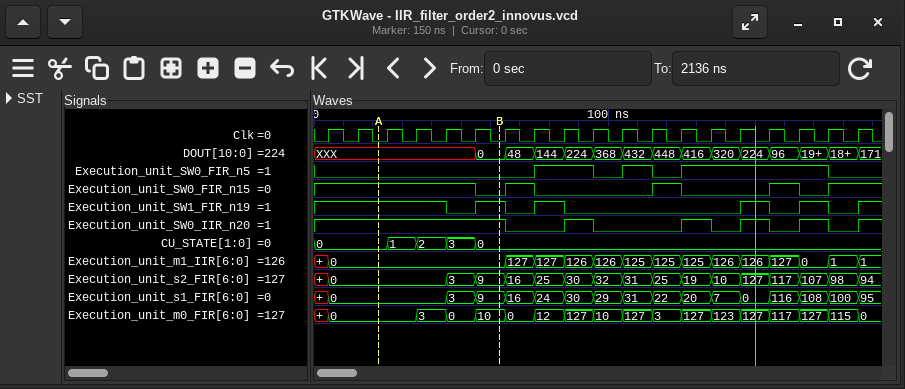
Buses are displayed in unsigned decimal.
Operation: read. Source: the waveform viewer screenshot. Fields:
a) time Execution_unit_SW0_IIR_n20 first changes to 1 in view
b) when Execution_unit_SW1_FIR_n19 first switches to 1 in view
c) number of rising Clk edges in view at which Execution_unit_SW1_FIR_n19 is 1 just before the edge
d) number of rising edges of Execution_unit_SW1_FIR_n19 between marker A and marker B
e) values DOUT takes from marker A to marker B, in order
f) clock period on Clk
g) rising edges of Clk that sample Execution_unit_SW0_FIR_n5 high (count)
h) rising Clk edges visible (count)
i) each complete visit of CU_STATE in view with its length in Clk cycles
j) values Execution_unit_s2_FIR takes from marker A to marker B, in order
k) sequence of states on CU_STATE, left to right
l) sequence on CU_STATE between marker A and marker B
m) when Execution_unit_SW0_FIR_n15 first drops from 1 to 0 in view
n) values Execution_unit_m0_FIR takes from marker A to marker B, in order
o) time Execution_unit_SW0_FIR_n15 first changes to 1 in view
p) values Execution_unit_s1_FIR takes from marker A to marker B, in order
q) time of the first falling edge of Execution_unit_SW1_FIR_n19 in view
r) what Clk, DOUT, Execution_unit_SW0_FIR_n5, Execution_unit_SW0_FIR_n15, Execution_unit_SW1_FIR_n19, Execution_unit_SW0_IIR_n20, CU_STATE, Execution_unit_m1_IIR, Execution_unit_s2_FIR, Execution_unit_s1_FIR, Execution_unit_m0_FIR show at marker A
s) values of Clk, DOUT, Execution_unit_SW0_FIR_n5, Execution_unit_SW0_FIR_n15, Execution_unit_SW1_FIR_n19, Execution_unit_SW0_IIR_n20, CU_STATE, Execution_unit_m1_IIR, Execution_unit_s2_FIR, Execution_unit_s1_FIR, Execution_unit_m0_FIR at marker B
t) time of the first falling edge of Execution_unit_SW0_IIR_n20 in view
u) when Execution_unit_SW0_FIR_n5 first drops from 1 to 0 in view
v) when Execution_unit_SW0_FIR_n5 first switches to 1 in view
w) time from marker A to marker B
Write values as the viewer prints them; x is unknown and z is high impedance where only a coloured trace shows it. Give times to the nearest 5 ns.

85 ns
55 ns
9
1
XXX, 0
10 ns
8
19
1: 1, 2: 1, 3: 1
0, 3, 9
0, 1, 2, 3, 0
0, 1, 2, 3, 0
55 ns
0, 3, 0, 10
65 ns
0, 3, 9
45 ns
Clk=0, DOUT=XXX, Execution_unit_SW0_FIR_n5=0, Execution_unit_SW0_FIR_n15=1, Execution_unit_SW1_FIR_n19=1, Execution_unit_SW0_IIR_n20=1, CU_STATE=0, Execution_unit_m1_IIR=0, Execution_unit_s2_FIR=0, Execution_unit_s1_FIR=0, Execution_unit_m0_FIR=0
Clk=0, DOUT=0, Execution_unit_SW0_FIR_n5=0, Execution_unit_SW0_FIR_n15=0, Execution_unit_SW1_FIR_n19=1, Execution_unit_SW0_IIR_n20=1, CU_STATE=0, Execution_unit_m1_IIR=0, Execution_unit_s2_FIR=9, Execution_unit_s1_FIR=9, Execution_unit_m0_FIR=10
65 ns
95 ns
75 ns
40 ns
